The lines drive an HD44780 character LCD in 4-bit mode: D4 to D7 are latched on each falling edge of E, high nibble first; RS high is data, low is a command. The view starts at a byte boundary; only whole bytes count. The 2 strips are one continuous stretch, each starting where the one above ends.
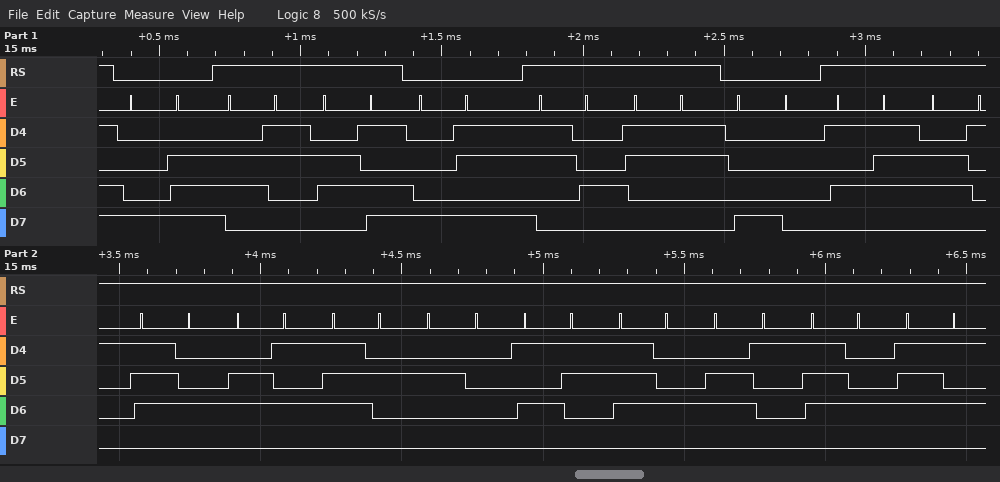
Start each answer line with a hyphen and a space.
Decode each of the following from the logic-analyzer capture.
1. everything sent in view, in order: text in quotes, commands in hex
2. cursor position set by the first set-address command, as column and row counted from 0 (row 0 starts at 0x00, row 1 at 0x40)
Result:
- 0x8E "cm" 0x8B "43" 0x80 "Water Statu"
- column 14, row 0
